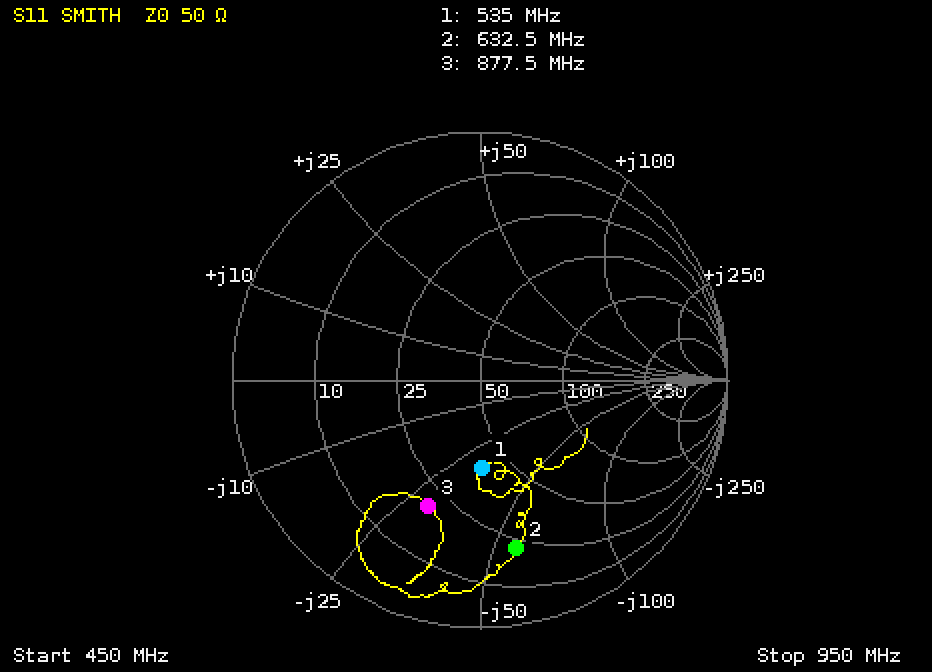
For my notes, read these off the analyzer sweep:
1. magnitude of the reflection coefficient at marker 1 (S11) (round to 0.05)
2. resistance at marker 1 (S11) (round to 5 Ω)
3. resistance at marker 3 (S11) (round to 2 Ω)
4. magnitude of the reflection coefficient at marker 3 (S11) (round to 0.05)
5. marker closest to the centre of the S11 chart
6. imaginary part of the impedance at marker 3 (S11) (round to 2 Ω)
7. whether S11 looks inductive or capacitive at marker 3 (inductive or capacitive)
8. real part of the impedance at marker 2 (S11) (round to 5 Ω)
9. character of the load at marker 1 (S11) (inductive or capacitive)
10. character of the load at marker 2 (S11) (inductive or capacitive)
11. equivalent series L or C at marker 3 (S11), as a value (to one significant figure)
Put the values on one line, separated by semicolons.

0.35; 40 Ω; 20 Ω; 0.55; marker 1; -30 Ω; capacitive; 20 Ω; capacitive; capacitive; 6 pF
